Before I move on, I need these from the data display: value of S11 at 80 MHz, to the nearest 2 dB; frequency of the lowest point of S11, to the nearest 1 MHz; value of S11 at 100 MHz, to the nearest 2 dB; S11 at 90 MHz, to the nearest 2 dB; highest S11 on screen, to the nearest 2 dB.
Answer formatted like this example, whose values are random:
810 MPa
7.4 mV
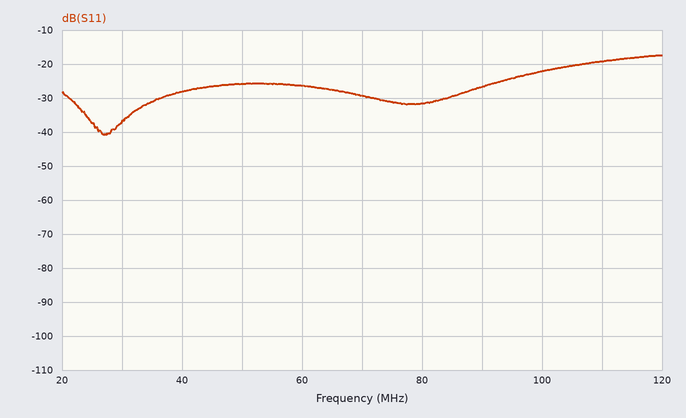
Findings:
-32 dB
27 MHz
-22 dB
-26 dB
-18 dB
